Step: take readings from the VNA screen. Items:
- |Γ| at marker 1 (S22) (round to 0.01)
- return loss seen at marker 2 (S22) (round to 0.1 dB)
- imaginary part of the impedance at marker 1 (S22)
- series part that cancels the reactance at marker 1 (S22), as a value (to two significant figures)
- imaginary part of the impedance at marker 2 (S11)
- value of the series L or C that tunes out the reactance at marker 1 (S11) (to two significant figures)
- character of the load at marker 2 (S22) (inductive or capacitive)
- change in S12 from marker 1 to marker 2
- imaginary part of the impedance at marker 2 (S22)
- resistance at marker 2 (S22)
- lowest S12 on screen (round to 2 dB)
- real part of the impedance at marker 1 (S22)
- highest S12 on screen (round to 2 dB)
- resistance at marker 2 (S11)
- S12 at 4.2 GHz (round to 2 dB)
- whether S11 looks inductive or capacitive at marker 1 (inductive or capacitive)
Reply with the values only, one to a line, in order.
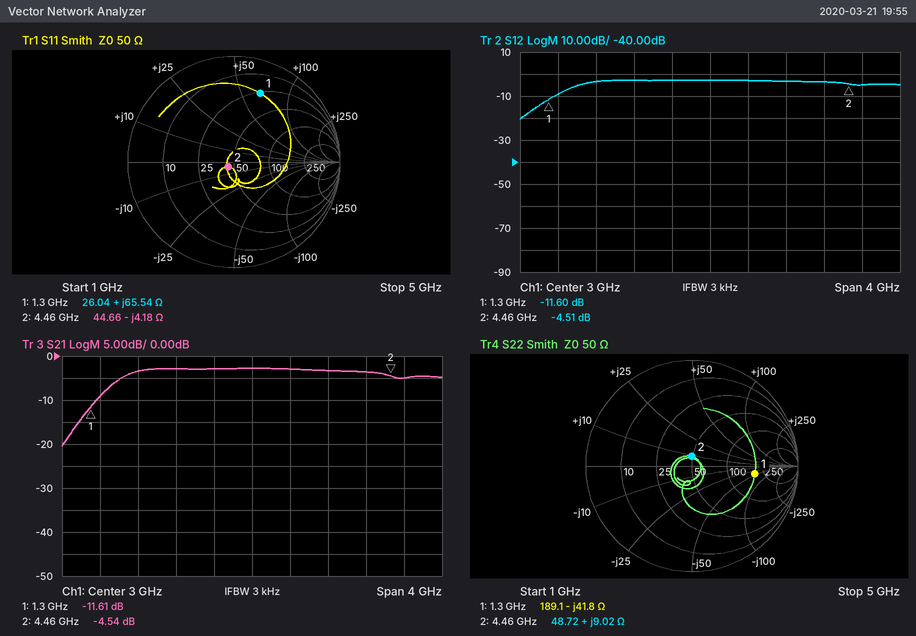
0.60
20.7 dB
-41.8 Ω
5.1 nH
-4.18 Ω
1.9 pF
inductive
7.09 dB
+9.02 Ω
48.72 Ω
-20 dB
189.1 Ω
-2 dB
44.66 Ω
-4 dB
inductive
